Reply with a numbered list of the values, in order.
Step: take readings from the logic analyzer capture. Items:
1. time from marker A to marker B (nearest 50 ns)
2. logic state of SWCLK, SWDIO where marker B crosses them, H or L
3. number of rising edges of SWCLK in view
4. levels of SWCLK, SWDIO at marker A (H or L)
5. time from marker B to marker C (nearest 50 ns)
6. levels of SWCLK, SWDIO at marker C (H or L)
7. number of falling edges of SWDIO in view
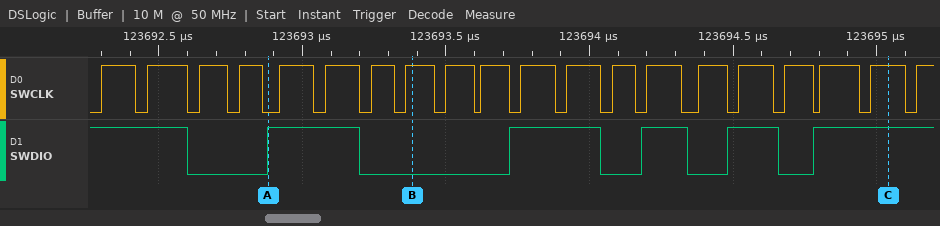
1. 500 ns
2. SWCLK=H, SWDIO=L
3. 20
4. SWCLK=L, SWDIO=H
5. 1650 ns
6. SWCLK=H, SWDIO=H
7. 5
